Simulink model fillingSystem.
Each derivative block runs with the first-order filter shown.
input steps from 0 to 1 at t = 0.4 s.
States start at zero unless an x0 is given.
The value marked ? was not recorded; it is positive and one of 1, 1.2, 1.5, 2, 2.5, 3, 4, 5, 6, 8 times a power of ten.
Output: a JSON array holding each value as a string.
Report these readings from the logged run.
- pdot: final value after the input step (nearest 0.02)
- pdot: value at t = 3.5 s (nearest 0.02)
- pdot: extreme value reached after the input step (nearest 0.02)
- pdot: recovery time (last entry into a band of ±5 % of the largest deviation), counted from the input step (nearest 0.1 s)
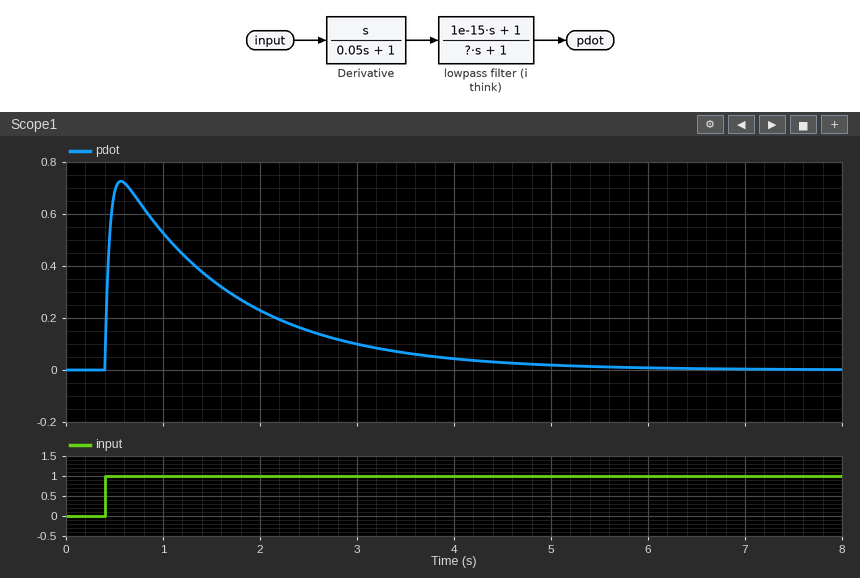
["0.00", "0.06", "0.72", "3.8 s"]
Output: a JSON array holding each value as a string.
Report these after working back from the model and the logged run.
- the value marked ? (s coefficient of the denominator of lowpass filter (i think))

["1.2"]
